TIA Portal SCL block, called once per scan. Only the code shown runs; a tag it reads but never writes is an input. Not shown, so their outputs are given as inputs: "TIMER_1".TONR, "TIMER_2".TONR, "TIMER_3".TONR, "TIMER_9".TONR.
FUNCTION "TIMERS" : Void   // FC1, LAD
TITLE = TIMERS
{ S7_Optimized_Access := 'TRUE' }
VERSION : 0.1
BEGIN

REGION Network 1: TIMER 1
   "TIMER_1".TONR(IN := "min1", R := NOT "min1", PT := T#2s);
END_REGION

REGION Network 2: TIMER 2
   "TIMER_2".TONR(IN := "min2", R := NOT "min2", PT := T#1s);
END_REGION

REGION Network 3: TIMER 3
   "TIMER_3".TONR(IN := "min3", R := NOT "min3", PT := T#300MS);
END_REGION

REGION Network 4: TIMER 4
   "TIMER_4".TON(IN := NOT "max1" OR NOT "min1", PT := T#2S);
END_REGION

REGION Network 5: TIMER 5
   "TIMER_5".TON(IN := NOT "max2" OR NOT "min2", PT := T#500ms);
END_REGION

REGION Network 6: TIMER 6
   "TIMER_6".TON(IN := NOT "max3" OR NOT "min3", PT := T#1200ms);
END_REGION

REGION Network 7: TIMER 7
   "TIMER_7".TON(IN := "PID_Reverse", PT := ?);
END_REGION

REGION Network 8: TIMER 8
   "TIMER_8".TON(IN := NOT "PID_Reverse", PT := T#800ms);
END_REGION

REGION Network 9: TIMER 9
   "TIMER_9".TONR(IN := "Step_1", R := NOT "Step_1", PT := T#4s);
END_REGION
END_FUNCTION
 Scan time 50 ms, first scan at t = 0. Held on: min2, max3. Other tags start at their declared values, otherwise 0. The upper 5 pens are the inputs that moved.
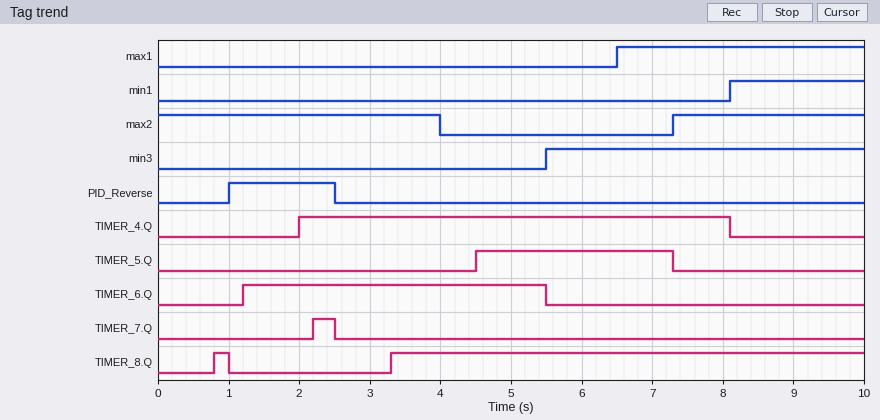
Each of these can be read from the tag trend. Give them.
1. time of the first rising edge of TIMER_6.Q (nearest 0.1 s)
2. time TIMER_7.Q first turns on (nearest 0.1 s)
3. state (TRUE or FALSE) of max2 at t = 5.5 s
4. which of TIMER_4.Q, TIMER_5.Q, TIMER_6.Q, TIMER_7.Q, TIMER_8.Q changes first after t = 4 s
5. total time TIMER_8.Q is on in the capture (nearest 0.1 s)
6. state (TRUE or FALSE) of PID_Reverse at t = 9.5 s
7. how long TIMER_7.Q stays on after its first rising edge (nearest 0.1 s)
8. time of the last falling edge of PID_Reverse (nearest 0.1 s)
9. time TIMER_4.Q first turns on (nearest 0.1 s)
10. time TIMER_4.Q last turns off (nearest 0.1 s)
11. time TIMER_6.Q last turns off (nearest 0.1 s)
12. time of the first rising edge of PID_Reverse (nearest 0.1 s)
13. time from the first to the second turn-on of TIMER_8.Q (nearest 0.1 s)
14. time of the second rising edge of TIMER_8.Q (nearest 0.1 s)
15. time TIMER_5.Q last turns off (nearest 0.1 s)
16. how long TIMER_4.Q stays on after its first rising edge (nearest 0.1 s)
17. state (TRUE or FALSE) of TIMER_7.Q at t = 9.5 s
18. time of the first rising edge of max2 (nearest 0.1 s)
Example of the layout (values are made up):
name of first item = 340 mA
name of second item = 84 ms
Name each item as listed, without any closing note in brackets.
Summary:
time of the first rising edge of TIMER_6.Q = 1.2 s
time TIMER_7.Q first turns on = 2.2 s
state (TRUE or FALSE) of max2 at t = 5.5 s = FALSE
which of TIMER_4.Q, TIMER_5.Q, TIMER_6.Q, TIMER_7.Q, TIMER_8.Q changes first after t = 4 s = TIMER_5.Q
total time TIMER_8.Q is on in the capture = 6.9 s
state (TRUE or FALSE) of PID_Reverse at t = 9.5 s = FALSE
how long TIMER_7.Q stays on after its first rising edge = 0.3 s
time of the last falling edge of PID_Reverse = 2.5 s
time TIMER_4.Q first turns on = 2.0 s
time TIMER_4.Q last turns off = 8.1 s
time TIMER_6.Q last turns off = 5.5 s
time of the first rising edge of PID_Reverse = 1.0 s
time from the first to the second turn-on of TIMER_8.Q = 2.5 s
time of the second rising edge of TIMER_8.Q = 3.3 s
time TIMER_5.Q last turns off = 7.3 s
how long TIMER_4.Q stays on after its first rising edge = 6.1 s
state (TRUE or FALSE) of TIMER_7.Q at t = 9.5 s = FALSE
time of the first rising edge of max2 = 7.3 s
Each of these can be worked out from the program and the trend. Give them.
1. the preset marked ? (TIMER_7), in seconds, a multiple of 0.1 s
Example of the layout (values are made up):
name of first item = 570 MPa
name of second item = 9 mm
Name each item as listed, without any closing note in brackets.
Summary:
the preset marked ? (TIMER_7), in seconds, a multiple of 0.1 s = 1.2 s
